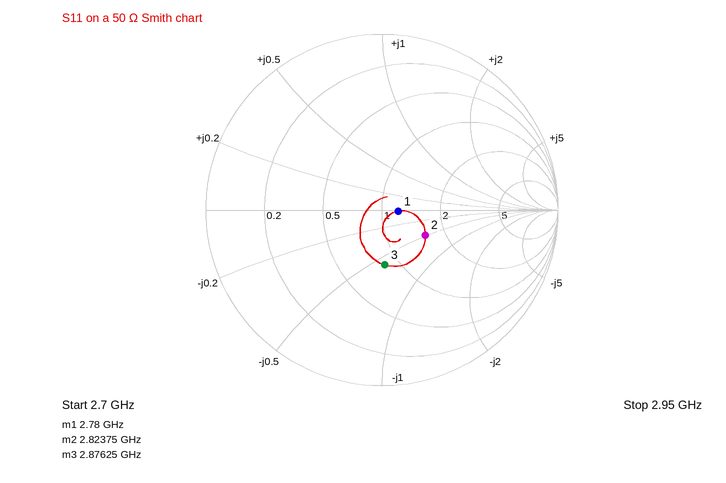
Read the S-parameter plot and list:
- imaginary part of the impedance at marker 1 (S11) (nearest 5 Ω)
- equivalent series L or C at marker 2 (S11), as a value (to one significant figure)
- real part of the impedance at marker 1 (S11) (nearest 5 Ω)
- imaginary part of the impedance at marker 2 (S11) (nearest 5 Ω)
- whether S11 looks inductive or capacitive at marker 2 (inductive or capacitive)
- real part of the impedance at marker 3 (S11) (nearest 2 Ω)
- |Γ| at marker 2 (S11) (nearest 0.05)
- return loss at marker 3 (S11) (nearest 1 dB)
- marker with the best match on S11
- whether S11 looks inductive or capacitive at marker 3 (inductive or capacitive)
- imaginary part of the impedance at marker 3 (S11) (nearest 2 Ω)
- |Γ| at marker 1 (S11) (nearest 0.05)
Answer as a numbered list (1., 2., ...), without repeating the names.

1. 0 Ω
2. 2 pF
3. 60 Ω
4. -25 Ω
5. capacitive
6. 42 Ω
7. 0.30
8. 10 dB
9. marker 1
10. capacitive
11. -30 Ω
12. 0.10
